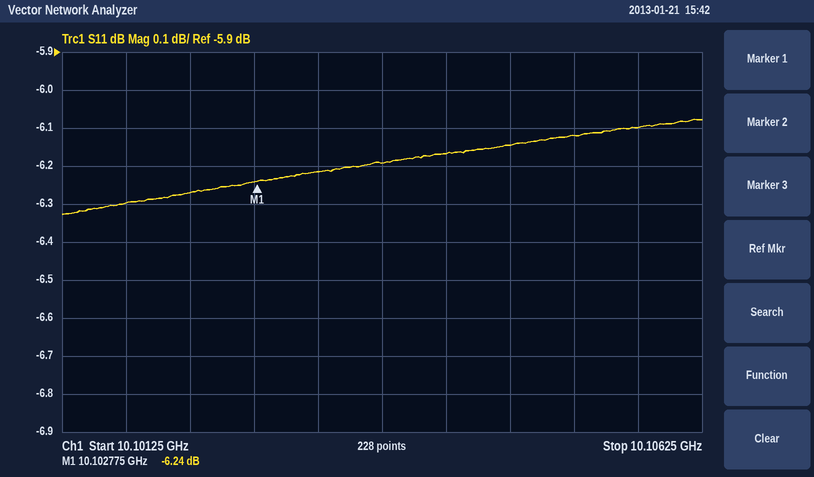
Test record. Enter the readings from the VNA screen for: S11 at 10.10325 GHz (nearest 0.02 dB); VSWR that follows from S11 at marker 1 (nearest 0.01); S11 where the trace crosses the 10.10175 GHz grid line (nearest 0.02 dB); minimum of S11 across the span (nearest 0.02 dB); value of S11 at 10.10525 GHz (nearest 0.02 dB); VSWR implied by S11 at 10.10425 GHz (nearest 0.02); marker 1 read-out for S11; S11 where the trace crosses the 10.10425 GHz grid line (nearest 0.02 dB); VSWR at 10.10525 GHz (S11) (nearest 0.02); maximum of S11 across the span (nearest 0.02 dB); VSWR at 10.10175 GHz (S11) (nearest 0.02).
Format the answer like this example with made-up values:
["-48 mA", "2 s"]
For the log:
["-6.22 dB", "2.90", "-6.30 dB", "-6.32 dB", "-6.12 dB", "2.94", "-6.24 dB", "-6.16 dB", "2.96", "-6.08 dB", "2.88"]
